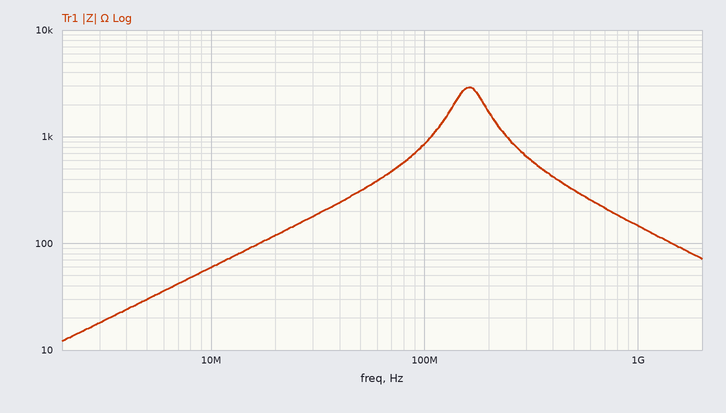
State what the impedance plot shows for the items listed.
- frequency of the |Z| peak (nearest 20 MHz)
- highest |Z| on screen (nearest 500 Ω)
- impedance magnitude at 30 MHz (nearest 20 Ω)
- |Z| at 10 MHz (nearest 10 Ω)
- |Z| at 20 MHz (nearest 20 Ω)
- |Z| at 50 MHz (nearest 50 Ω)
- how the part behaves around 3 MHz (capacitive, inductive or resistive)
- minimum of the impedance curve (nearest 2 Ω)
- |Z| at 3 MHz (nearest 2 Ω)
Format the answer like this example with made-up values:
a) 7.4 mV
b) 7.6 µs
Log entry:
a) 160 MHz
b) 3.0 kΩ
c) 180 Ω
d) 60 Ω
e) 120 Ω
f) 300 Ω
g) inductive
h) 12 Ω
i) 18 Ω
